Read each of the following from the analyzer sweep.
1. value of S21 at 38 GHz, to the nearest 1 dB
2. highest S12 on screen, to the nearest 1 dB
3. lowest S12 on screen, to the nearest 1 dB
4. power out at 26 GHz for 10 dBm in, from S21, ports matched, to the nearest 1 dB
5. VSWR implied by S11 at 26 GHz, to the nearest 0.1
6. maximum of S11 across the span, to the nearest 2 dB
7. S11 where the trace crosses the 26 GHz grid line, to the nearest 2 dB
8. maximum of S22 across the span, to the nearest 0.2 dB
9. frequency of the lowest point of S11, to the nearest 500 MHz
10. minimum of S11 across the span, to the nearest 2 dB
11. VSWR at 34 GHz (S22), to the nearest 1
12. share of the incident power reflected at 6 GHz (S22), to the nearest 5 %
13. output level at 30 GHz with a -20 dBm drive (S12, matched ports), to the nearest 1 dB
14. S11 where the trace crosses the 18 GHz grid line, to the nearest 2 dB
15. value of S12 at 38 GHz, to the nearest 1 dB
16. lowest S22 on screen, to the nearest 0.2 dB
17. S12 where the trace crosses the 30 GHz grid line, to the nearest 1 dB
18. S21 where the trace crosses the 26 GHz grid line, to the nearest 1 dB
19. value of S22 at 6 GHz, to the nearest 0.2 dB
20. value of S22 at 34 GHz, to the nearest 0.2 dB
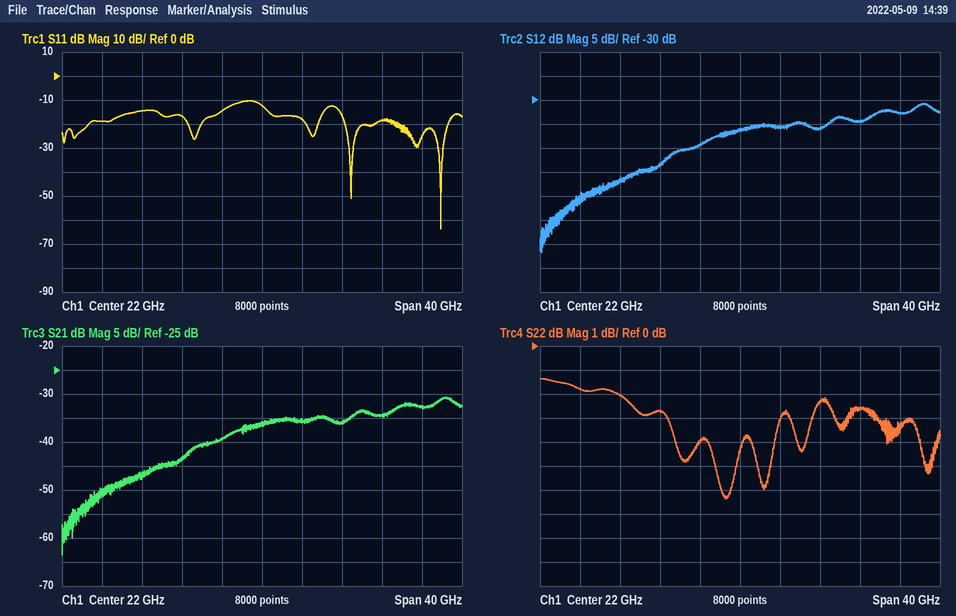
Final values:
-33 dB
-31 dB
-62 dB
-26 dBm
1.3
-10 dB
-18 dB
-1.4 dB
40.0 GHz
-64 dB
7
65 %
-56 dBm
-14 dB
-33 dB
-6.4 dB
-36 dB
-36 dB
-1.8 dB
-2.6 dB
